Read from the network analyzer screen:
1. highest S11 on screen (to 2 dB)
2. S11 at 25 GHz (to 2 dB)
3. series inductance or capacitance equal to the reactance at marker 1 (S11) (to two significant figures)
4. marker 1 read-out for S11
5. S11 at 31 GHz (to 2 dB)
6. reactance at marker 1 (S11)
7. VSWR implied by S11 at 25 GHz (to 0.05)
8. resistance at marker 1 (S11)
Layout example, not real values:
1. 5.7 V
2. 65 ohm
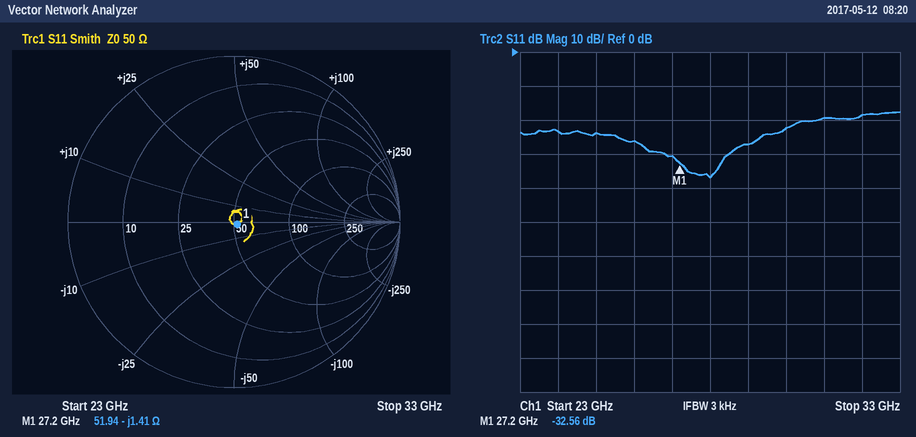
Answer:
1. -18 dB
2. -24 dB
3. 4.1 pF
4. -32.56 dB
5. -20 dB
6. -1.41 Ω
7. 1.15
8. 51.94 Ω
